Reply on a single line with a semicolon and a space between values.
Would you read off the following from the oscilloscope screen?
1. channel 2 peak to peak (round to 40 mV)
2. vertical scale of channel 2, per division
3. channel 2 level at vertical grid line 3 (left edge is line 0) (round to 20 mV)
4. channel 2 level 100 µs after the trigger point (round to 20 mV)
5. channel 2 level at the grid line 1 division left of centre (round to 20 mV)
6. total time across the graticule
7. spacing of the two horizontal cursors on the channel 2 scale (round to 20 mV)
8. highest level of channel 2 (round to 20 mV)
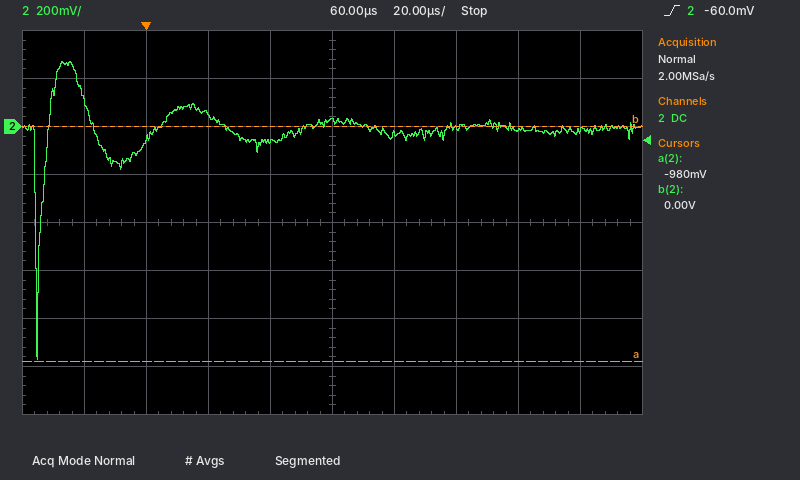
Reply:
1.24 V; 200 mV; 40 mV; 0 mV; -60 mV; 200 µs; 980 mV; 280 mV
